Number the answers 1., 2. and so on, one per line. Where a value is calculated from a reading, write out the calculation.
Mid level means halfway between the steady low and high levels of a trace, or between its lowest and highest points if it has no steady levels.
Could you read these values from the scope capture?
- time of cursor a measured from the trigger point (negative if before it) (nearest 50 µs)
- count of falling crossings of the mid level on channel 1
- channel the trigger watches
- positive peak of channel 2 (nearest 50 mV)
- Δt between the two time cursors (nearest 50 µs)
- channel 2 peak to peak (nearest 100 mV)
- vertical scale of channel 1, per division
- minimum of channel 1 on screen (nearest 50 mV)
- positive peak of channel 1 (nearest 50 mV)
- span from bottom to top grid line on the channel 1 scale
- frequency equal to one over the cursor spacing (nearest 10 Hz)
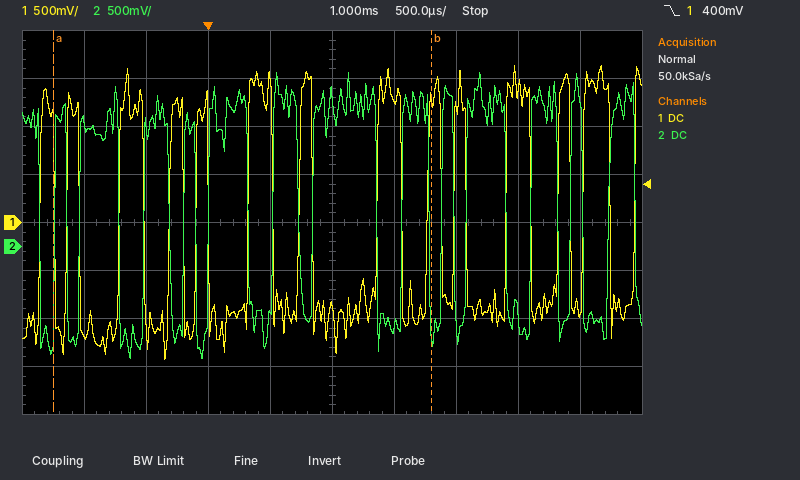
1. -1.25 ms
2. 13
3. channel 1
4. 1.80 V
5. 3.05 ms
6. 3.00 V
7. 500 mV
8. -1.45 V
9. 1.65 V
10. 4 V
11. 1 / 3.05 ms ≈ 330 Hz
